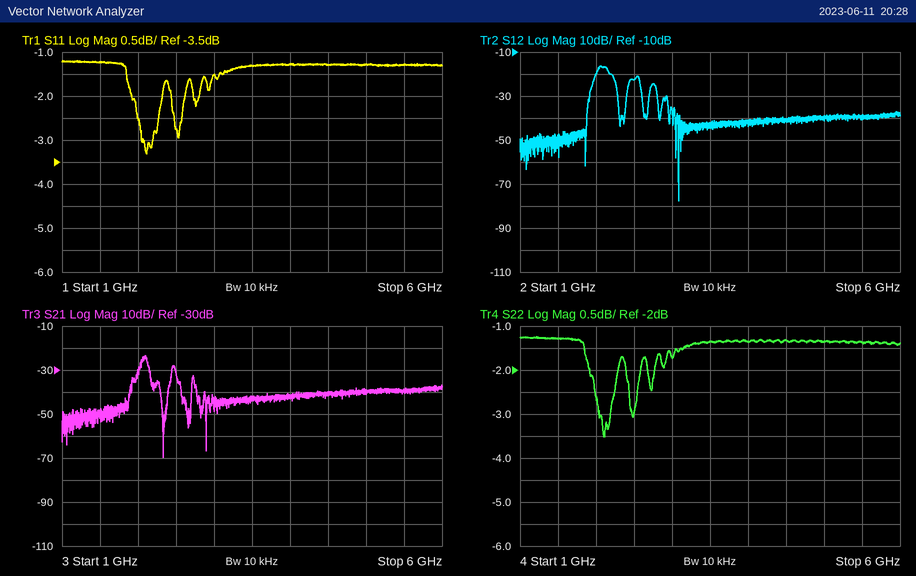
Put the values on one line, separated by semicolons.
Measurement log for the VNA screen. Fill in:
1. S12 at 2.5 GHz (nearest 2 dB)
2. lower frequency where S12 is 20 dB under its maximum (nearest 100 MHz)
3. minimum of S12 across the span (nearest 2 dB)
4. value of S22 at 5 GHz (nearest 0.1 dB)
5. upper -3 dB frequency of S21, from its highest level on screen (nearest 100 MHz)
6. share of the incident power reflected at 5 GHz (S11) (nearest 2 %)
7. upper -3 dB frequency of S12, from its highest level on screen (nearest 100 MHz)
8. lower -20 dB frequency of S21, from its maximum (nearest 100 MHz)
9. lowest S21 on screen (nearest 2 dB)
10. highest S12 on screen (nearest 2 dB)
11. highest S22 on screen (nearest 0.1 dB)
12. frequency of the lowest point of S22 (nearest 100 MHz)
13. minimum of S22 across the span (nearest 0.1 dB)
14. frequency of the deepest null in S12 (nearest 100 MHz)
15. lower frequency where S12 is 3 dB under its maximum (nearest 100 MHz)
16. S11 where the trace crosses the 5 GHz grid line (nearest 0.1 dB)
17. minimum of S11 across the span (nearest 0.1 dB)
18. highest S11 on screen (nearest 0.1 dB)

-22 dB; 1.9 GHz; -78 dB; -1.4 dB; 2.1 GHz; 74 %; 2.2 GHz; 1.9 GHz; -70 dB; -16 dB; -1.2 dB; 2.1 GHz; -3.5 dB; 3.1 GHz; 2.0 GHz; -1.3 dB; -3.3 dB; -1.2 dB
